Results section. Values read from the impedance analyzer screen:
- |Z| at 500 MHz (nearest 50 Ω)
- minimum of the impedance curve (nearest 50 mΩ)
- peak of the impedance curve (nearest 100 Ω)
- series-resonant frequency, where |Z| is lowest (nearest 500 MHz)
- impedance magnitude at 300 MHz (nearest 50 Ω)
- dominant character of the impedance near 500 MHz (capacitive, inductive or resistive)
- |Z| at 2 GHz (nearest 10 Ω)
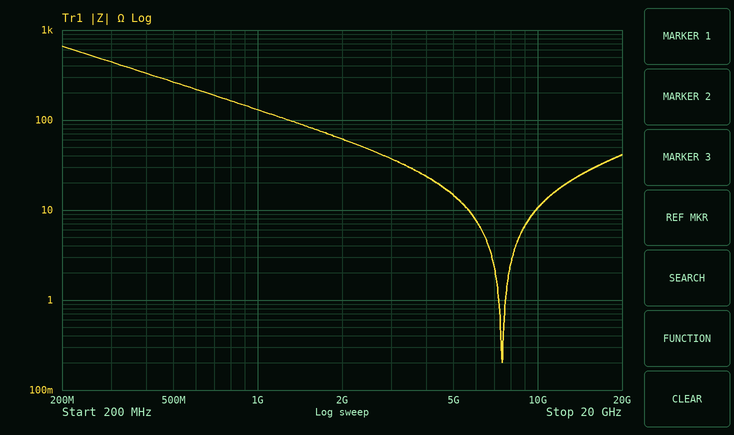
250 Ω
200 mΩ
700 Ω
7.5 GHz
450 Ω
capacitive
60 Ω
